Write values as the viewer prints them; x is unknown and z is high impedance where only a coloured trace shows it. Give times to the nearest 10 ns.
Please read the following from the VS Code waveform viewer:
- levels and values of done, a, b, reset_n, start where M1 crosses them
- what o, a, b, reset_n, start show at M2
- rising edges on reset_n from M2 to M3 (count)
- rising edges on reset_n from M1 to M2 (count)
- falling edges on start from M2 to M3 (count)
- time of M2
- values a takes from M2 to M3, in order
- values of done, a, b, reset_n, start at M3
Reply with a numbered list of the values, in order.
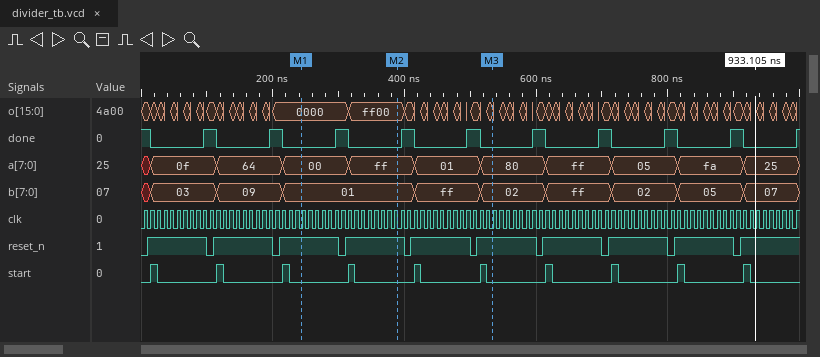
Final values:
1. done=0, a=00, b=01, reset_n=1, start=0
2. o=ff00, a=ff, b=01, reset_n=1, start=0
3. 2
4. 1
5. 2
6. 390 ns
7. ff, 01, 80
8. done=0, a=80, b=02, reset_n=1, start=0
